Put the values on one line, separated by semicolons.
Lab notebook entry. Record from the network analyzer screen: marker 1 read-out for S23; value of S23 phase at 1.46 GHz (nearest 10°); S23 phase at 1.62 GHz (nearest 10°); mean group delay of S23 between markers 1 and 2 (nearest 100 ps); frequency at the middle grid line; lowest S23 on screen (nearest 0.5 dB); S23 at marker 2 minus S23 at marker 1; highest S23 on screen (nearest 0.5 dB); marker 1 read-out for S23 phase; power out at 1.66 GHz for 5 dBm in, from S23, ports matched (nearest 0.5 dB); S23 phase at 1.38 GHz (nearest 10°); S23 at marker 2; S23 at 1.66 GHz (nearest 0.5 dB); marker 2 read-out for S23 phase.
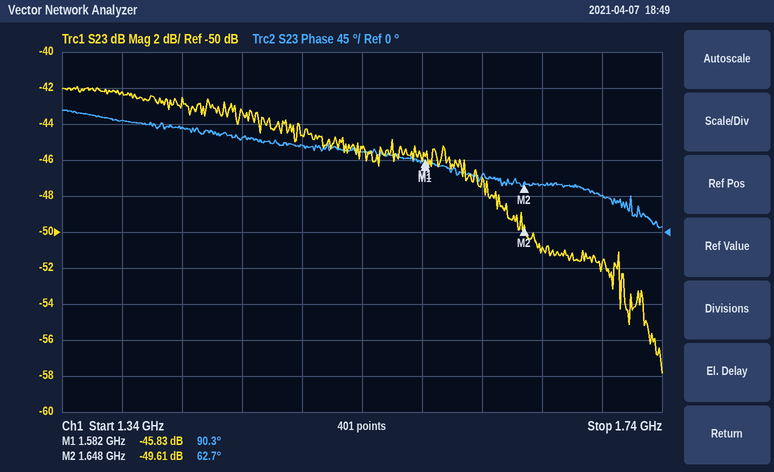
-45.83 dB; 120°; 70°; 1.2 ns; 1.54 GHz; -58.0 dB; -3.78 dB; -42.0 dB; 90.3°; -46.0 dBm; 140°; -49.61 dB; -51.0 dB; 62.7°
